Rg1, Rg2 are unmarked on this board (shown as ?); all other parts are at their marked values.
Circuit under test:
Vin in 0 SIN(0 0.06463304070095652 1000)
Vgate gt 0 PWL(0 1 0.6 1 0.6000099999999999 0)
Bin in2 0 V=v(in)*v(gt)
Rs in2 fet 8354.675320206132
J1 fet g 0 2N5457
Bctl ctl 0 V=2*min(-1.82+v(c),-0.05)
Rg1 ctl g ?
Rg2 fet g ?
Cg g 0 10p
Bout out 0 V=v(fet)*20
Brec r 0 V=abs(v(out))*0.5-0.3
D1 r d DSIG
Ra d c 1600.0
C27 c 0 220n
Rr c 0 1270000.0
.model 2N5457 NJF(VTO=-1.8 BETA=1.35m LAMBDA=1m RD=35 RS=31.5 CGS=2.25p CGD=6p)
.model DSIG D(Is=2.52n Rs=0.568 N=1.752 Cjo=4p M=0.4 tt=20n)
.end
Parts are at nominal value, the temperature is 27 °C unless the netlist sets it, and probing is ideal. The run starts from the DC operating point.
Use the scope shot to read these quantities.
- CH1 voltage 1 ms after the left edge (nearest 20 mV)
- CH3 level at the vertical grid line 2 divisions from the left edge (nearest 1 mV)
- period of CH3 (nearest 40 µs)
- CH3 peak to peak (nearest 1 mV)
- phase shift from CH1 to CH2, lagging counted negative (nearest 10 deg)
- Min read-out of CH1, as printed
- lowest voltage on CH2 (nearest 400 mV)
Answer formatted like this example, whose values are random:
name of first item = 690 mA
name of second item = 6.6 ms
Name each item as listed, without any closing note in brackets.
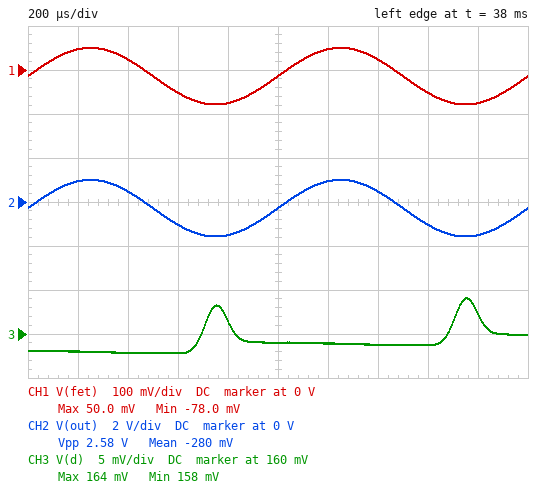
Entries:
CH1 voltage 1 ms after the left edge = -20 mV
CH3 level at the vertical grid line 2 divisions from the left edge = 158 mV
period of CH3 = 1.00 ms
CH3 peak to peak = 6 mV
phase shift from CH1 to CH2, lagging counted negative = 0 deg
Min read-out of CH1, as printed = -78.0 mV
lowest voltage on CH2 = -1.6 V
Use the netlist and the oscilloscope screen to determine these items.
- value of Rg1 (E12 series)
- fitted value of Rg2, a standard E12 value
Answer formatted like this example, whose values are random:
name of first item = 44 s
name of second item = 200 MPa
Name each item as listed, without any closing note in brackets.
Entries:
value of Rg1 = 470 kΩ
fitted value of Rg2, a standard E12 value = 1.5 MΩ
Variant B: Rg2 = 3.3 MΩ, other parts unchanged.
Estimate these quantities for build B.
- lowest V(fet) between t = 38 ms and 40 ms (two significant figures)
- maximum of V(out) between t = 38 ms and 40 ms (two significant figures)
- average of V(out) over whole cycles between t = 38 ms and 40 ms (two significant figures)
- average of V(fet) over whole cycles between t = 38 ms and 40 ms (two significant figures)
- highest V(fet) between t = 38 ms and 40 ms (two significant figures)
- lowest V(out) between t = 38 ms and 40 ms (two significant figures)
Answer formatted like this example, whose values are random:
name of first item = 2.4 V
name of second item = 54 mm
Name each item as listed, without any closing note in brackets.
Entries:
lowest V(fet) between t = 38 ms and 40 ms = -72 mV
maximum of V(out) between t = 38 ms and 40 ms = 1.1 V
average of V(out) over whole cycles between t = 38 ms and 40 ms = -150 mV
average of V(fet) over whole cycles between t = 38 ms and 40 ms = -7.6 mV
highest V(fet) between t = 38 ms and 40 ms = 57 mV
lowest V(out) between t = 38 ms and 40 ms = -1.4 V
